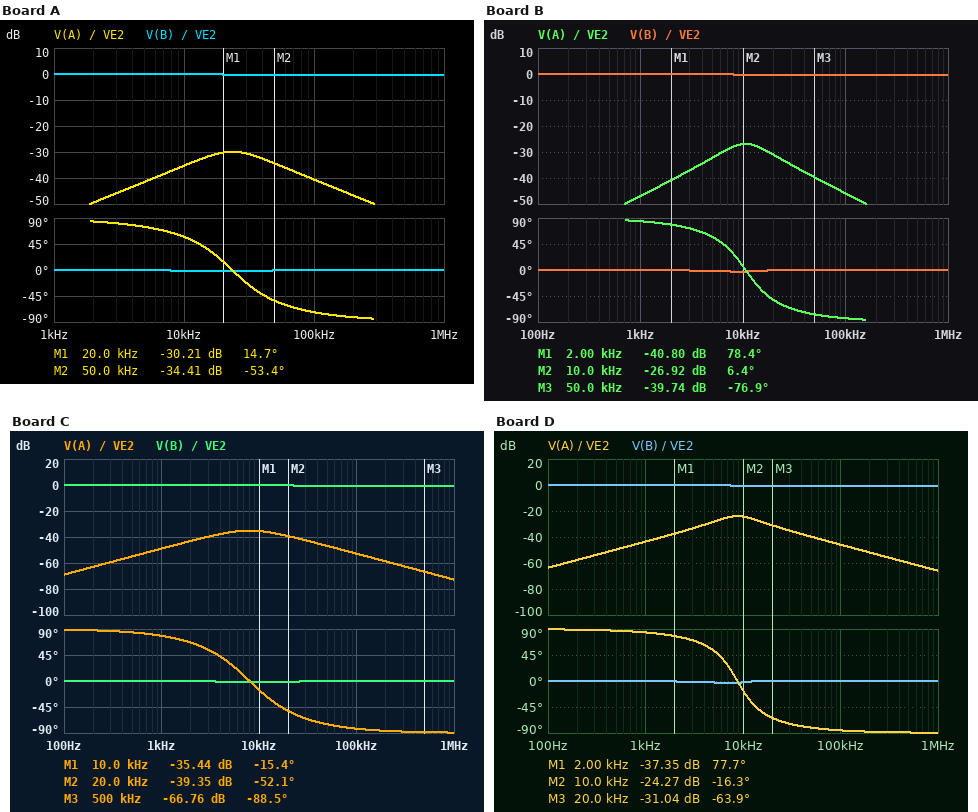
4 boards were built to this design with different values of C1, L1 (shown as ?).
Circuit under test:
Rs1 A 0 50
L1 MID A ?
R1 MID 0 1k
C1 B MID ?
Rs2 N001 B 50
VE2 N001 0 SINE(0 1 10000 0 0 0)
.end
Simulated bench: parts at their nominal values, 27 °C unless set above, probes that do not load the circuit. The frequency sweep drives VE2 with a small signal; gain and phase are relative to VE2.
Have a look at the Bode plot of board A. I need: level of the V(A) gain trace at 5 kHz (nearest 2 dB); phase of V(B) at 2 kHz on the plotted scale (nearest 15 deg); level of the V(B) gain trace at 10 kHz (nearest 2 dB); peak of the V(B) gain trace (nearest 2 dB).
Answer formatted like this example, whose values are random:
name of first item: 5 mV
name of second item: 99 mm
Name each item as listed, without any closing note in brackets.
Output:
level of the V(A) gain trace at 5 kHz: -42 dB
phase of V(B) at 2 kHz on the plotted scale: 0 deg
level of the V(B) gain trace at 10 kHz: 0 dB
peak of the V(B) gain trace: 0 dB
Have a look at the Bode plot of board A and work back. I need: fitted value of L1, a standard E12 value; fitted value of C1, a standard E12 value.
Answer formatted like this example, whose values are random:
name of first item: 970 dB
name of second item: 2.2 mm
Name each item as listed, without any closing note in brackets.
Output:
fitted value of L1, a standard E12 value: 8.2 mH
fitted value of C1, a standard E12 value: 5.6 nF
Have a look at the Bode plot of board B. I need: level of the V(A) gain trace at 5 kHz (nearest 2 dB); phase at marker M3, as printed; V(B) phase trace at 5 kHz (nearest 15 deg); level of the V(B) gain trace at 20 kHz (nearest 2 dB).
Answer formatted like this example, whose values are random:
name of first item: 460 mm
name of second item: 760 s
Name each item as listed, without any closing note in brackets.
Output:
level of the V(A) gain trace at 5 kHz: -32 dB
phase at marker M3, as printed: -76.9 deg
V(B) phase trace at 5 kHz: 0 deg
level of the V(B) gain trace at 20 kHz: 0 dB
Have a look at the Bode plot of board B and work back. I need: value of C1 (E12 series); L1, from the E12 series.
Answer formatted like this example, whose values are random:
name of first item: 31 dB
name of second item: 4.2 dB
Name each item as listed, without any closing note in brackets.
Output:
value of C1: 15 nF
L1, from the E12 series: 15 mH
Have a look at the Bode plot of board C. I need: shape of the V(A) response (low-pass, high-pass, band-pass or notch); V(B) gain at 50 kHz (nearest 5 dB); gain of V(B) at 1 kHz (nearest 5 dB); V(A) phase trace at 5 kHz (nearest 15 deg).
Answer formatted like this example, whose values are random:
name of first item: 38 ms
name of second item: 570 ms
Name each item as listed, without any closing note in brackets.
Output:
shape of the V(A) response: band-pass
V(B) gain at 50 kHz: 0 dB
gain of V(B) at 1 kHz: 0 dB
V(A) phase trace at 5 kHz: 30 deg
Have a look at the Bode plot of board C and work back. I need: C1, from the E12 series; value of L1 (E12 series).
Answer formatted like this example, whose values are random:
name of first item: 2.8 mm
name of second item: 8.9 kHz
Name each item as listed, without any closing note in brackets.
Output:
C1, from the E12 series: 12 nF
value of L1: 33 mH
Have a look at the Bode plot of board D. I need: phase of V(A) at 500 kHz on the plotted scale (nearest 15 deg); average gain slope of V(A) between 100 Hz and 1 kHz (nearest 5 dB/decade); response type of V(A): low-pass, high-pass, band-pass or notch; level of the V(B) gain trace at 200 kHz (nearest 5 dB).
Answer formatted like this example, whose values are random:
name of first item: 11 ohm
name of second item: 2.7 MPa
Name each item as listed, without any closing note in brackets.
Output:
phase of V(A) at 500 kHz on the plotted scale: -90 deg
average gain slope of V(A) between 100 Hz and 1 kHz: 20 dB/decade
response type of V(A): low-pass, high-pass, band-pass or notch: band-pass
level of the V(B) gain trace at 200 kHz: 0 dB
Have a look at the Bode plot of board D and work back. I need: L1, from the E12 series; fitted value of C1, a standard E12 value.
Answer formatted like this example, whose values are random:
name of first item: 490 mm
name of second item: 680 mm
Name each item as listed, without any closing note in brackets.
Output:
L1, from the E12 series: 15 mH
fitted value of C1, a standard E12 value: 22 nF
